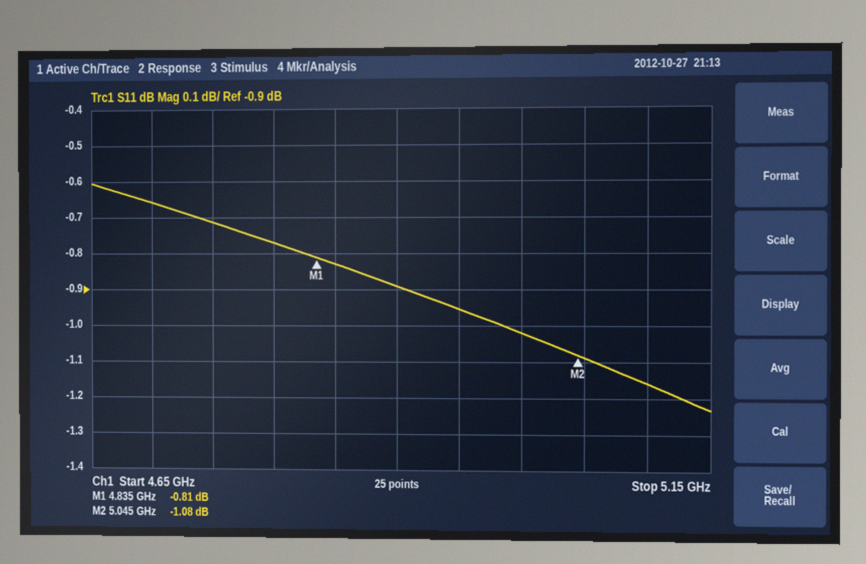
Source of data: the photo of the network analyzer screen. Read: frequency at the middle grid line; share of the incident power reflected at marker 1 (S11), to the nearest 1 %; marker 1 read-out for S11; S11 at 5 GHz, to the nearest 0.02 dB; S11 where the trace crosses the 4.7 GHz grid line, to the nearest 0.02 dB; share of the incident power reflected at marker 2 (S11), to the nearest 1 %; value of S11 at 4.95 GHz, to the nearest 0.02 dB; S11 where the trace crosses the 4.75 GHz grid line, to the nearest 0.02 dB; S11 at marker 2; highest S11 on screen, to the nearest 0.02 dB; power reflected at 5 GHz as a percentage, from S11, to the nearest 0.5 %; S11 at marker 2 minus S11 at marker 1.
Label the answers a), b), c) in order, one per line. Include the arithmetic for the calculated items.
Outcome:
a) 4.9 GHz
b) 10^(-0.81/10) ≈ 83 %
c) -0.81 dB
d) -1.02 dB
e) -0.66 dB
f) 10^(-1.08/10) ≈ 78 %
g) -0.96 dB
h) -0.72 dB
i) -1.08 dB
j) -0.60 dB
k) 10^(-1.02/10) ≈ 79.1 %, so 79.0 % to the nearest 0.5 %
l) -1.08 − (-0.81) = -0.27 dB
